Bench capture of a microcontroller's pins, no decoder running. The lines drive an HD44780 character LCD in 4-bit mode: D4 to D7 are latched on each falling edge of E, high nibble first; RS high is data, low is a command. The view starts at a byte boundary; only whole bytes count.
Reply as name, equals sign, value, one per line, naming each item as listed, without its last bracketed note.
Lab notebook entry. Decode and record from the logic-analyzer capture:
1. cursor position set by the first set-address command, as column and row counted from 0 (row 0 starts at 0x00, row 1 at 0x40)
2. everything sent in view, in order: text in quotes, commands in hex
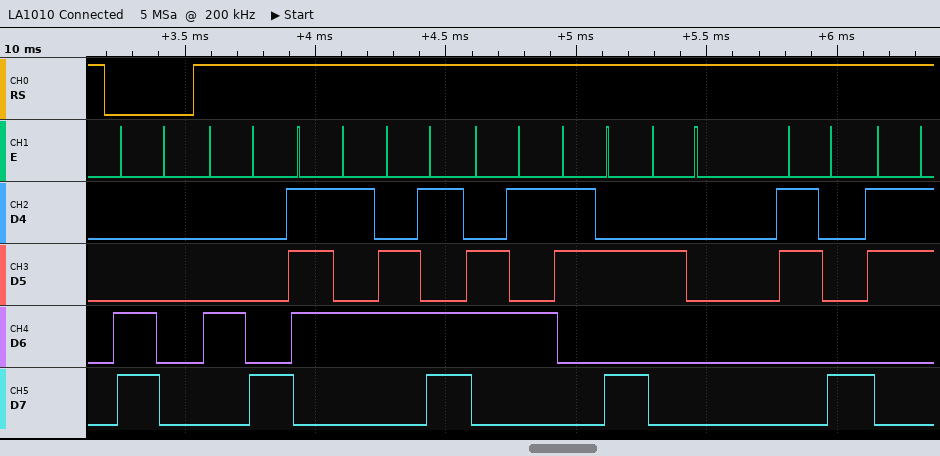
cursor position set by the first set-address command, as column and row counted from 0 = column 0, row 1
everything sent in view, in order: text in quotes, commands in hex = 0xC0 "Hume: 83"
